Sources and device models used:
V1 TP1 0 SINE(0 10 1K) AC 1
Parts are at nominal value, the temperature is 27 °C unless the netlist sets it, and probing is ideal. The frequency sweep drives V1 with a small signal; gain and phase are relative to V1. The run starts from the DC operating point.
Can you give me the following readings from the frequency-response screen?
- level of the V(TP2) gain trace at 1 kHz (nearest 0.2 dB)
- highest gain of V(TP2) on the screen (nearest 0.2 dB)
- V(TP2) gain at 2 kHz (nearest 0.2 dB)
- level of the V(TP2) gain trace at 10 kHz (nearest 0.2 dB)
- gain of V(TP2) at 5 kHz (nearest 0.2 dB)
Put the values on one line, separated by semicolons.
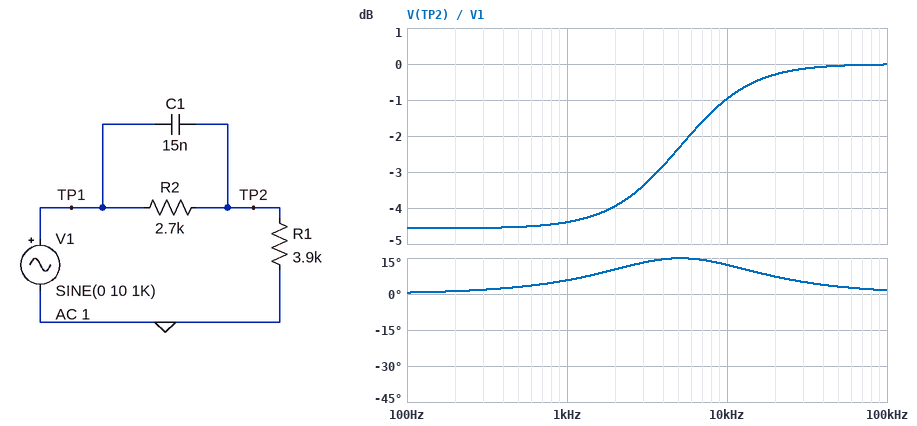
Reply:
-4.4 dB; 0 dB; -4.0 dB; -1.0 dB; -2.4 dB
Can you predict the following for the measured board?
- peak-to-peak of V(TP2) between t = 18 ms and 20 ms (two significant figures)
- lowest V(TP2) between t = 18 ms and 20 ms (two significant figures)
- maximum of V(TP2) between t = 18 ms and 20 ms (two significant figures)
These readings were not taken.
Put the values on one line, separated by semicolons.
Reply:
12 V; -6.0 V; 6.0 V
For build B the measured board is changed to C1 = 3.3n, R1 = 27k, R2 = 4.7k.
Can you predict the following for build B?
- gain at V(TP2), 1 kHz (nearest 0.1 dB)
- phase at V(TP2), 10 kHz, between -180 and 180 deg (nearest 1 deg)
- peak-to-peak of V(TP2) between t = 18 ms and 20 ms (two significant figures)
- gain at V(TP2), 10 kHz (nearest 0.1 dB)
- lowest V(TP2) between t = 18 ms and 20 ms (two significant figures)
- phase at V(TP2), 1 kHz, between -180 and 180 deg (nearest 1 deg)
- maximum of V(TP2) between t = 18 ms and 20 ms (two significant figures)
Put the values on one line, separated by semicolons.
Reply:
-1.4 dB; 5 deg; 17 V; -0.8 dB; -8.5 V; 1 deg; 8.5 V
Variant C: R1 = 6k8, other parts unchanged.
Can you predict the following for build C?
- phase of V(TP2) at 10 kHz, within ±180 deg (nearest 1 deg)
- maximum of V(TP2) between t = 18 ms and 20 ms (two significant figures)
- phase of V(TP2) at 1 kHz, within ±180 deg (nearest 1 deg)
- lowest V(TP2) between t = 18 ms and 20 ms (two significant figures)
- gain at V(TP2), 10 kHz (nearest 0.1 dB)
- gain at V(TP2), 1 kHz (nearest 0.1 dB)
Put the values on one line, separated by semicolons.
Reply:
7 deg; 7.3 V; 4 deg; -7.3 V; -0.5 dB; -2.8 dB
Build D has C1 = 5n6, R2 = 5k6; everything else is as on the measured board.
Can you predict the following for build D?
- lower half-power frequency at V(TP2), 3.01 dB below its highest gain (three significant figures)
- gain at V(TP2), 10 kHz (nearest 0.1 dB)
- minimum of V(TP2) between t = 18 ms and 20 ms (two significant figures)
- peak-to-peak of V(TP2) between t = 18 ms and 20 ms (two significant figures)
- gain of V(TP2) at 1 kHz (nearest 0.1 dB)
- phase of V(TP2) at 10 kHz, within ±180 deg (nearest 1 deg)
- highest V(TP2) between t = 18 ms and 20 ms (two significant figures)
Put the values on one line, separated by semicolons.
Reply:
10.1 kHz; -3.0 dB; -4.2 V; 8.3 V; -7.6 dB; 24 deg; 4.2 V
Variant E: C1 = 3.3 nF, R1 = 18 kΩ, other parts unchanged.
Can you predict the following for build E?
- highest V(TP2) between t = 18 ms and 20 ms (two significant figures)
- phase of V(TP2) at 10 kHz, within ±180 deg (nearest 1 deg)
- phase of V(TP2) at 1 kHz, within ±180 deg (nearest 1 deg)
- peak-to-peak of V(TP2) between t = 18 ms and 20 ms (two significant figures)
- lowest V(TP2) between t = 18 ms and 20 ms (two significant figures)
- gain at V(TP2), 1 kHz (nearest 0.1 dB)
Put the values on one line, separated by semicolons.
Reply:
8.7 V; 3 deg; 0 deg; 17 V; -8.7 V; -1.2 dB
